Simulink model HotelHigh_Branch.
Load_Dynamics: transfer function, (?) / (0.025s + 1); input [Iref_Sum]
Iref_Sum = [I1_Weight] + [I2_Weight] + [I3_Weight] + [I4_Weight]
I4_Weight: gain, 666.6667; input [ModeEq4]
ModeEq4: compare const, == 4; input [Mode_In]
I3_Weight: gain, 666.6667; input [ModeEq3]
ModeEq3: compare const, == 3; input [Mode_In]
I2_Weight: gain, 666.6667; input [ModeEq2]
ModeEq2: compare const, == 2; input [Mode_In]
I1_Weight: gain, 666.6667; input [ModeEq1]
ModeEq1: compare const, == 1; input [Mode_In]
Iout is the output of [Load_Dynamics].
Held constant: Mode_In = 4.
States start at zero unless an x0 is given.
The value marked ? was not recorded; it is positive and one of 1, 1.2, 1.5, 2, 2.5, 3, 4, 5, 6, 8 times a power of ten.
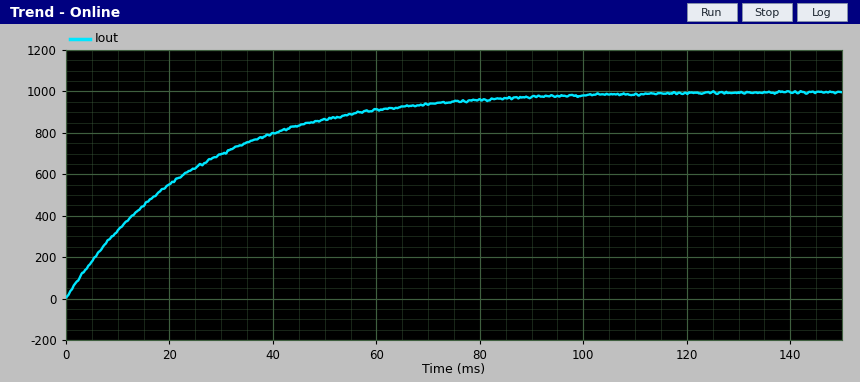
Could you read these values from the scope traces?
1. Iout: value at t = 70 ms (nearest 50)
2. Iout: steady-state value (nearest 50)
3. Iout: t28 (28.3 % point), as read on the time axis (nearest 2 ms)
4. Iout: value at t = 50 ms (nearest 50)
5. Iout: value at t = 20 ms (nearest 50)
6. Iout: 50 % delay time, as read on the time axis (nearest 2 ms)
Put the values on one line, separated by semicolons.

950; 1000; 8 ms; 850; 550; 18 ms
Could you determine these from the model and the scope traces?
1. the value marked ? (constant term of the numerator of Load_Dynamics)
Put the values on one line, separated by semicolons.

1.5
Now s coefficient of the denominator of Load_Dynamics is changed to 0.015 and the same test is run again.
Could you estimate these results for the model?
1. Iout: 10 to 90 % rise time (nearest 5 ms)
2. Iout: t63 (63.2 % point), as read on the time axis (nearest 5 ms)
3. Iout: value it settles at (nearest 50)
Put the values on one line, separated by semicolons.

35 ms; 15 ms; 1000
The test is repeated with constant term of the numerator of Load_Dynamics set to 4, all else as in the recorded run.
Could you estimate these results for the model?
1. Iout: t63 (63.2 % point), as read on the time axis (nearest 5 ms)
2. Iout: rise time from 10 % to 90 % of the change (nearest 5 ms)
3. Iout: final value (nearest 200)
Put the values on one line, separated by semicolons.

25 ms; 55 ms; 2600
